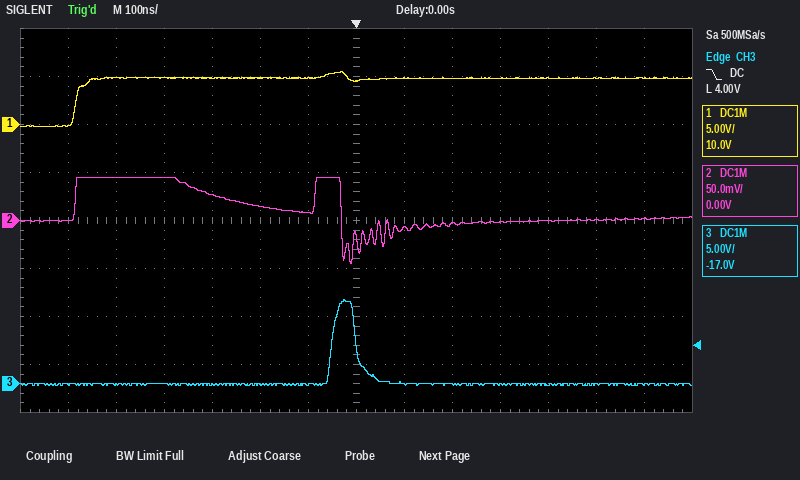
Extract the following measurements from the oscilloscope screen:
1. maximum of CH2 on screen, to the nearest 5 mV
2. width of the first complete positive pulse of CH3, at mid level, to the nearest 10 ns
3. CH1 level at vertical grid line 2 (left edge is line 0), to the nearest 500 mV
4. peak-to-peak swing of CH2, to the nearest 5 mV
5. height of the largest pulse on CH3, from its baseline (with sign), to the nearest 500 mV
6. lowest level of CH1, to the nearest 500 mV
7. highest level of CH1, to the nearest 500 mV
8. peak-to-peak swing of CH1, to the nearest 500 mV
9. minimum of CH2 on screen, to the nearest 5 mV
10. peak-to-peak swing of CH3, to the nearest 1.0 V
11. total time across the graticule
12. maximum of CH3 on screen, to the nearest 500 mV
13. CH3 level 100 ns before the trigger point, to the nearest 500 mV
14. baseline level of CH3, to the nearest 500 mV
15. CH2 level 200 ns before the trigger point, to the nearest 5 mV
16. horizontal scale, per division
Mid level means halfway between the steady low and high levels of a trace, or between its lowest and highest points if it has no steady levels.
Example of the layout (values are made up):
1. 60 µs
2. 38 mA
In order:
1. 45 mV
2. 50 ns
3. 5.0 V
4. 90 mV
5. +9.0 V
6. 0.0 V
7. 5.5 V
8. 5.5 V
9. -45 mV
10. 9.0 V
11. 1.4 µs
12. 9.0 V
13. 0.0 V
14. 0.0 V
15. 15 mV
16. 100 ns
